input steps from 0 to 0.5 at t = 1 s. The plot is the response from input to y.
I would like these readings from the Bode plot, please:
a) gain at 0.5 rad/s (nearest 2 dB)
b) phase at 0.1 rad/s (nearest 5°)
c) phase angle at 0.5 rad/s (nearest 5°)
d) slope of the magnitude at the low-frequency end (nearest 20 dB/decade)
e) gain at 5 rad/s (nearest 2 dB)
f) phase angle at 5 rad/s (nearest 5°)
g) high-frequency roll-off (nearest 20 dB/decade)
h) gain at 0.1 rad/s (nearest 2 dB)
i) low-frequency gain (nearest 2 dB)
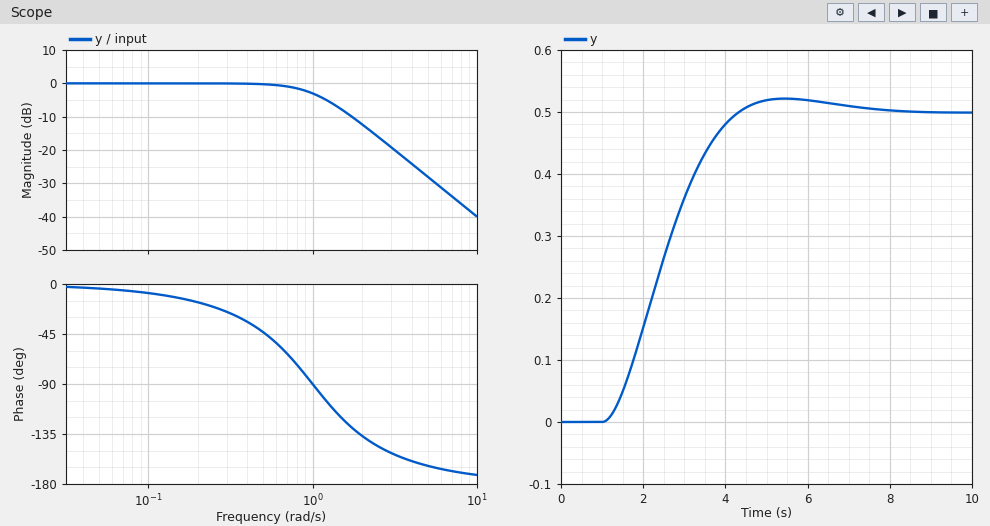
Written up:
0 dB
-10°
-45°
0 dB/decade
-28 dB
-165°
-40 dB/decade
0 dB
0 dB
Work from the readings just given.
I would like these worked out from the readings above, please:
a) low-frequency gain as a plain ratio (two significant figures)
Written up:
1.0
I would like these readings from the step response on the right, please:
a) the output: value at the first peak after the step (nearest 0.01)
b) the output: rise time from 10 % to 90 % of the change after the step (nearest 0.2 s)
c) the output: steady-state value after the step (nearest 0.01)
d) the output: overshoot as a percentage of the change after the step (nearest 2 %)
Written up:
0.52
2.2 s
0.50
4 %
